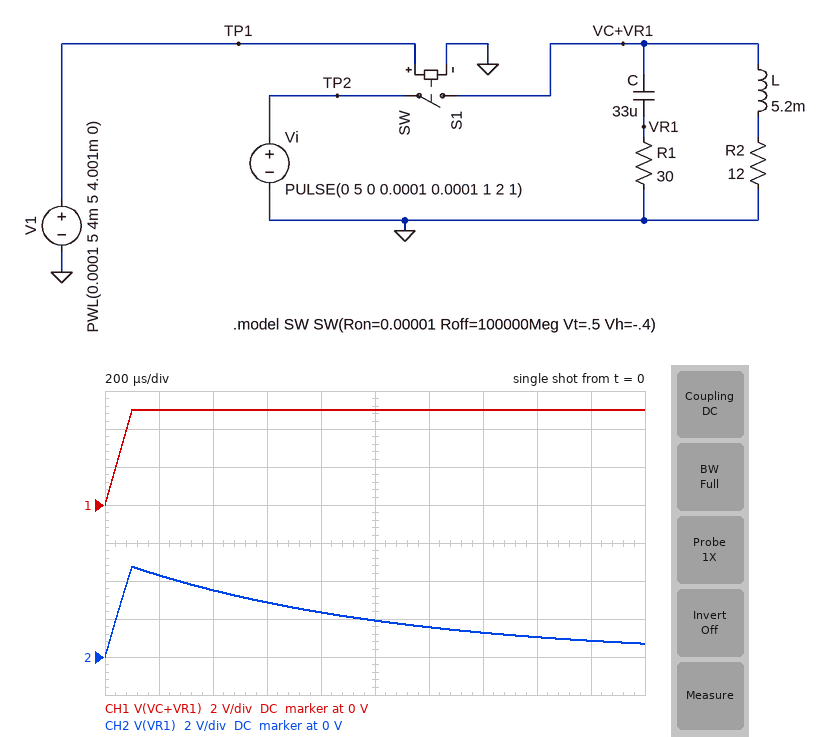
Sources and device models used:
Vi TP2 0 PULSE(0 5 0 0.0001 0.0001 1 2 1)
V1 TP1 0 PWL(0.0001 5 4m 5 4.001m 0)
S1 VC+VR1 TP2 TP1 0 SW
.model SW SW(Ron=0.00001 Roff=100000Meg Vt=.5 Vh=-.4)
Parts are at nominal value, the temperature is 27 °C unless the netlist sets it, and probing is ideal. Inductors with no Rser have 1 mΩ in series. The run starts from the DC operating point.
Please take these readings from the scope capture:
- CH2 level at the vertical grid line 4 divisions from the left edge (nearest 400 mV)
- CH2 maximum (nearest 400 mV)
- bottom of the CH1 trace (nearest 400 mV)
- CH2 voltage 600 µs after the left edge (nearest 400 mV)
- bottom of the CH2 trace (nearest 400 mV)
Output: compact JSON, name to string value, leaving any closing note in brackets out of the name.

{"CH2 level at the vertical grid line 4 divisions from the left edge": "2.4 V", "CH2 maximum": "4.8 V", "bottom of the CH1 trace": "0 V", "CH2 voltage 600 µs after the left edge": "2.8 V", "bottom of the CH2 trace": "0 V"}
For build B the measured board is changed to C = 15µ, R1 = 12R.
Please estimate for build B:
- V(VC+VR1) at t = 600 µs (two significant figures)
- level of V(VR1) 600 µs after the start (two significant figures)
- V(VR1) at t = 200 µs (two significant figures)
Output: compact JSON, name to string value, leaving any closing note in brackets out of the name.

{"V(VC+VR1) at t = 600 µs": "5.0 V", "level of V(VR1) 600 µs after the start": "240 mV", "V(VR1) at t = 200 µs": "2.2 V"}
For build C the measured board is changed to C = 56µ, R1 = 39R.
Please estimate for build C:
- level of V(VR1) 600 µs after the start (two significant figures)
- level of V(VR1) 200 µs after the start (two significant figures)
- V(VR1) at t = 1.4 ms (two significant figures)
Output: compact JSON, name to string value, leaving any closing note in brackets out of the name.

{"level of V(VR1) 600 µs after the start": "3.9 V", "level of V(VR1) 200 µs after the start": "4.7 V", "V(VR1) at t = 1.4 ms": "2.7 V"}
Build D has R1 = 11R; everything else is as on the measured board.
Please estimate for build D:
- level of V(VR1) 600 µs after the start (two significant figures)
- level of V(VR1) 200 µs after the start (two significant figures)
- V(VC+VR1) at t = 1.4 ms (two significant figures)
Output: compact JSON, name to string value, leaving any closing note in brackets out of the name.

{"level of V(VR1) 600 µs after the start": "1.1 V", "level of V(VR1) 200 µs after the start": "3.3 V", "V(VC+VR1) at t = 1.4 ms": "5.0 V"}
